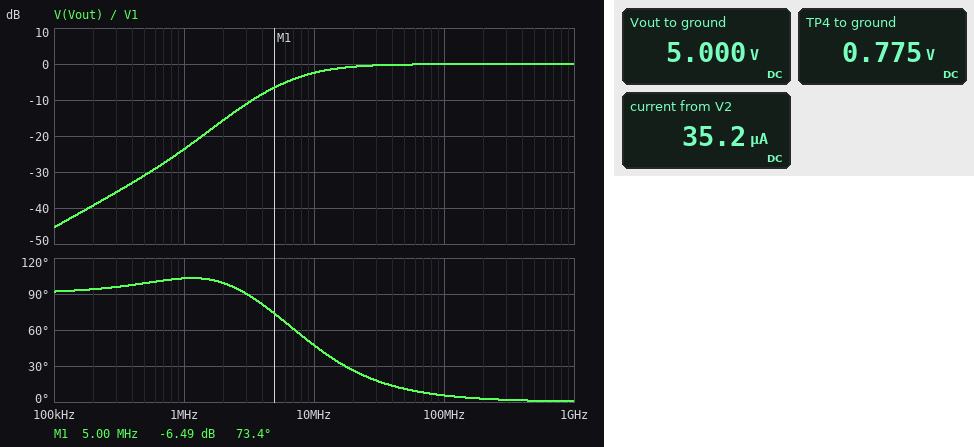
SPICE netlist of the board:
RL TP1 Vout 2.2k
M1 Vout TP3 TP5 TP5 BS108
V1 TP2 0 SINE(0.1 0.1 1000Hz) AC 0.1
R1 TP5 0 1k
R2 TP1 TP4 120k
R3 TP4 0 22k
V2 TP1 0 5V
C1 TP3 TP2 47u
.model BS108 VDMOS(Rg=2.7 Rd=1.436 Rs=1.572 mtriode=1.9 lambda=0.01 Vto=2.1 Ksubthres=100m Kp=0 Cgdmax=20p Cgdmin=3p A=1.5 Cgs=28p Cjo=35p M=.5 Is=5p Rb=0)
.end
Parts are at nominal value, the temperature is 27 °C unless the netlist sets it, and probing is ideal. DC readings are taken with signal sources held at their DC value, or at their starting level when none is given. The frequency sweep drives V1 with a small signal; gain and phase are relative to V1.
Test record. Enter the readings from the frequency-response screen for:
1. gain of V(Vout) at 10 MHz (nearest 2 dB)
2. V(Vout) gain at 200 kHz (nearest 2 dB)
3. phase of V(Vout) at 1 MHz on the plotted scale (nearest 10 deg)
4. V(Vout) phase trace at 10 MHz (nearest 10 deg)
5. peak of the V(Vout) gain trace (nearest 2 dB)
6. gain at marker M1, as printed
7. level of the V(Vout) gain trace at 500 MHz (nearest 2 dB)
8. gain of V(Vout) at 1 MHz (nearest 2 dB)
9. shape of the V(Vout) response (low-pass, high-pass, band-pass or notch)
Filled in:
-2 dB
-40 dB
100 deg
50 deg
0 dB
-6.49 dB
0 dB
-24 dB
high-pass
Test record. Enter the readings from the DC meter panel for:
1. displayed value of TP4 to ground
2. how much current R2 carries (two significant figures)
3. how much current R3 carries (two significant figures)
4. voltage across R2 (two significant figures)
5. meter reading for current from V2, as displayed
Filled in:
0.775 V
35 µA
35 µA
4.2 V
35.2 µA
